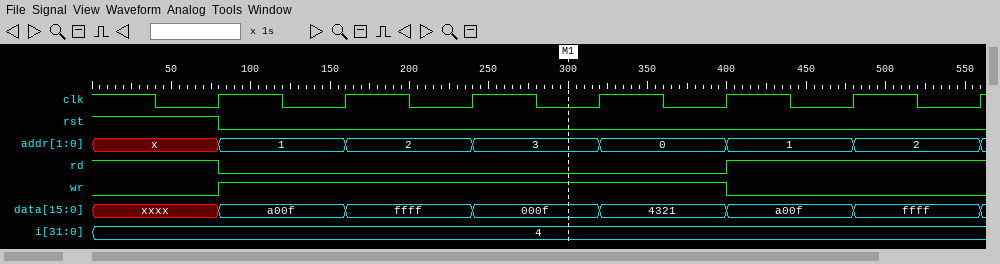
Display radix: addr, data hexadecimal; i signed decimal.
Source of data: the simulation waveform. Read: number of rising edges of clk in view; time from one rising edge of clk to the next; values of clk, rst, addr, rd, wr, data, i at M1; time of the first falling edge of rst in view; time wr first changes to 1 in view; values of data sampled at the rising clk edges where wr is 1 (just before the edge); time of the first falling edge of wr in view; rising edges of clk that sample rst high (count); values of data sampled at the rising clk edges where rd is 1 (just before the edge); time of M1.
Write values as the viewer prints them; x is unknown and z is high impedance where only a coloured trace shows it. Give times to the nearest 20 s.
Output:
7
80 s
clk=0, rst=0, addr=3, rd=0, wr=1, data=000f, i=4
80 s
80 s
a00f, ffff, 000f, 4321
400 s
1
xxxx, a00f, ffff
300 s
